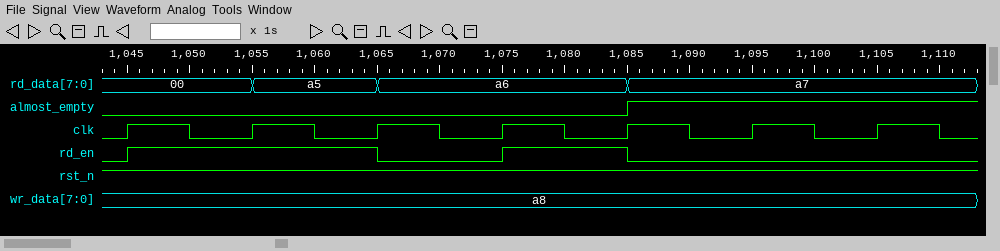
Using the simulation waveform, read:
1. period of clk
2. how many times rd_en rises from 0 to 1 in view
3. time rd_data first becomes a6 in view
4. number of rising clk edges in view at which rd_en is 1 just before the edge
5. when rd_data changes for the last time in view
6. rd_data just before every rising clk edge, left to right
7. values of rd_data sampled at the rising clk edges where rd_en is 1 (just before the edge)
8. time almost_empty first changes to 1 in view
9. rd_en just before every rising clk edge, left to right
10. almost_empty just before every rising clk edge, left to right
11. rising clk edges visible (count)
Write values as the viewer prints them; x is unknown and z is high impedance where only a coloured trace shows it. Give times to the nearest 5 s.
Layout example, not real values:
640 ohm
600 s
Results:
10 s
2
1065 s
3
1085 s
00, 00, a5, a6, a6, a7, a7
00, a5, a6
1085 s
0 1 1 0 1 0 0
0 0 0 0 0 1 1
7
